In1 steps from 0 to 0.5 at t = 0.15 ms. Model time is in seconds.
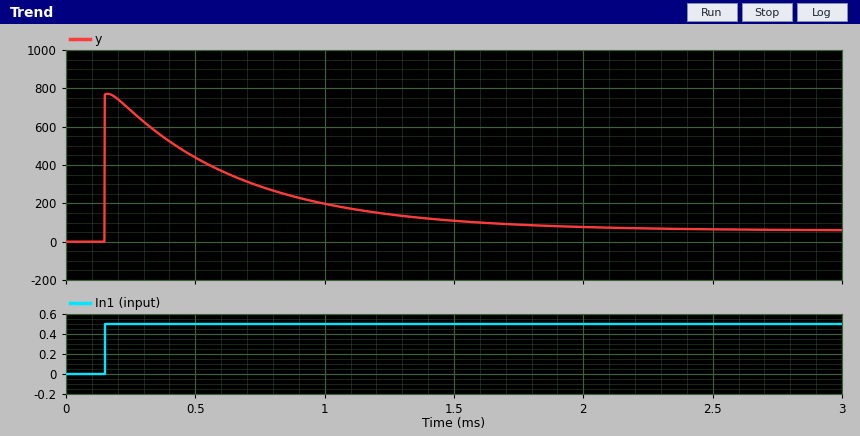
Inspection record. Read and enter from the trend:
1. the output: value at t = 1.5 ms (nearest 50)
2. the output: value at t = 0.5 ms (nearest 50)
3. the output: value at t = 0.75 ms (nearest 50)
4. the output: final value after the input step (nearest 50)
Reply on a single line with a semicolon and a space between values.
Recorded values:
100; 450; 300; 50
